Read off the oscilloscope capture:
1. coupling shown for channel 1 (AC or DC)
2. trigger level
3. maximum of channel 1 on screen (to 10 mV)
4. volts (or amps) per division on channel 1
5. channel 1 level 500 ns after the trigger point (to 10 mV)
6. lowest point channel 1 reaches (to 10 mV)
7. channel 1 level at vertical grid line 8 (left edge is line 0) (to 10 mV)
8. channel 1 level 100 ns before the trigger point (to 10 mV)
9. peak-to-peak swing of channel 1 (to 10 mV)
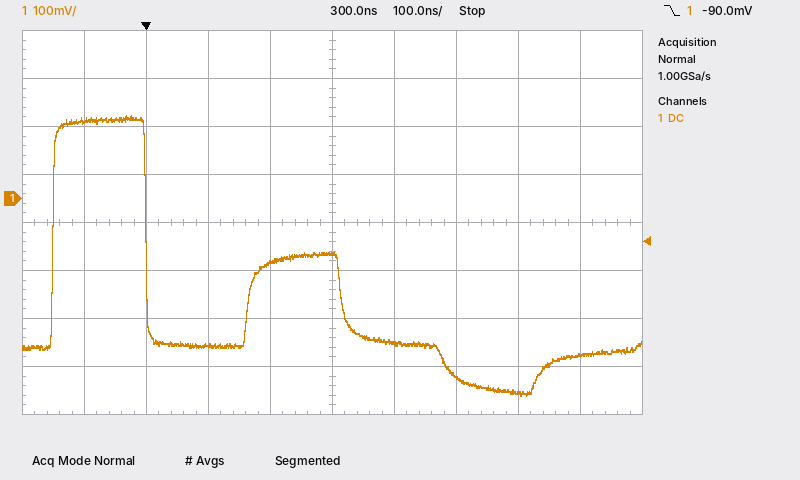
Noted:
DC
-90.0 mV
170 mV
100 mV
-370 mV
-410 mV
-410 mV
160 mV
580 mV
